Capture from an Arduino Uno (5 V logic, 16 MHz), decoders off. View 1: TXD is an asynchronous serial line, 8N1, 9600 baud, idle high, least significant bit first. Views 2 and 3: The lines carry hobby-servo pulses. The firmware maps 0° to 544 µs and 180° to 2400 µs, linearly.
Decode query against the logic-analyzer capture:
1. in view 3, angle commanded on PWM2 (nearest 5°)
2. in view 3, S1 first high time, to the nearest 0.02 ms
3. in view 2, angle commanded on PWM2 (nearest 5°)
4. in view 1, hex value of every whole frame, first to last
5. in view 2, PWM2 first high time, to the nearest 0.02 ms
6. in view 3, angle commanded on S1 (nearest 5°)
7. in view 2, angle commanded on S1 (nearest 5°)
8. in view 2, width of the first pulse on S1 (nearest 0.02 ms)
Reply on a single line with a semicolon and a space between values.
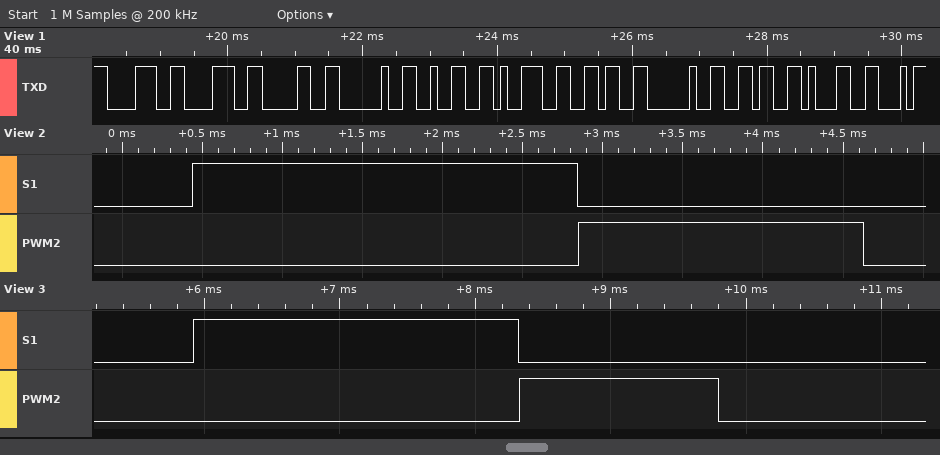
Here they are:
90°; 2.40 ms; 120°; 38 38 30 20 32 39 36 20 36 31; 1.78 ms; 180°; 180°; 2.40 ms
